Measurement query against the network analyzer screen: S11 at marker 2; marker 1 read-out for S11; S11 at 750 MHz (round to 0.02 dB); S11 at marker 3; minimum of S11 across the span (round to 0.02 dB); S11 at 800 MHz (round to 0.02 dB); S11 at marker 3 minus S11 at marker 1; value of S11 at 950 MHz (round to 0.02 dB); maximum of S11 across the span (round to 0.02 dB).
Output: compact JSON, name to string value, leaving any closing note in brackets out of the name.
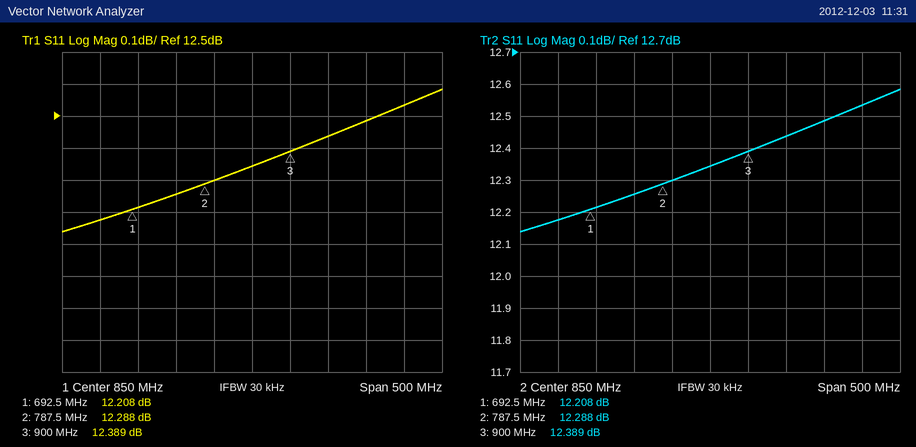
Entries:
{"S11 at marker 2": "12.288 dB", "marker 1 read-out for S11": "12.208 dB", "S11 at 750 MHz": "12.26 dB", "S11 at marker 3": "12.389 dB", "minimum of S11 across the span": "12.14 dB", "S11 at 800 MHz": "12.30 dB", "S11 at marker 3 minus S11 at marker 1": "0.181 dB", "value of S11 at 950 MHz": "12.44 dB", "maximum of S11 across the span": "12.58 dB"}
